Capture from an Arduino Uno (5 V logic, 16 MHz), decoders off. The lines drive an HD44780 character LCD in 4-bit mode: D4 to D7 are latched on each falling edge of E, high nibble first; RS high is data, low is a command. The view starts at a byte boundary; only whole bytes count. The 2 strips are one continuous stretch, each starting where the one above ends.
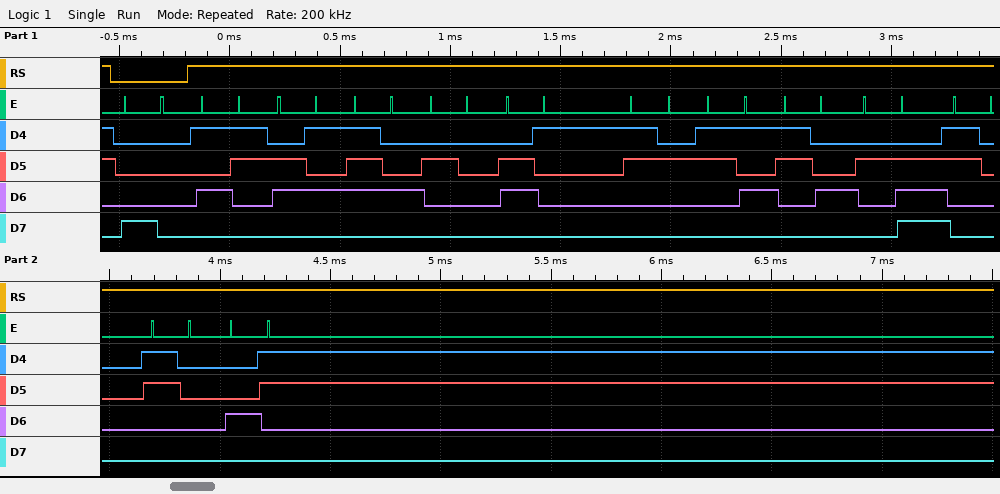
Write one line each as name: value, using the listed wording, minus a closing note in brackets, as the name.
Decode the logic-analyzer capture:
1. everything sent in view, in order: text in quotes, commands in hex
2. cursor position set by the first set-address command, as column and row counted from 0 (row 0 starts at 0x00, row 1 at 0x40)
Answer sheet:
everything sent in view, in order: text in quotes, commands in hex: 0x80 "Set a254.00C"
cursor position set by the first set-address command, as column and row counted from 0: column 0, row 0
